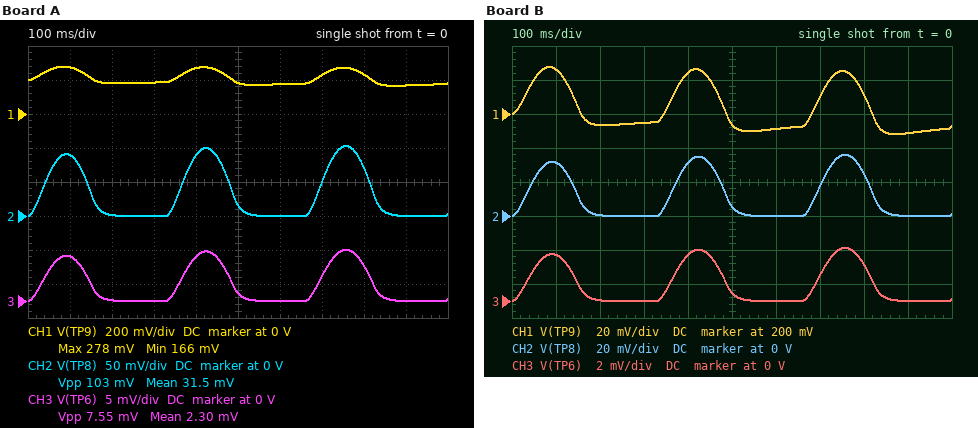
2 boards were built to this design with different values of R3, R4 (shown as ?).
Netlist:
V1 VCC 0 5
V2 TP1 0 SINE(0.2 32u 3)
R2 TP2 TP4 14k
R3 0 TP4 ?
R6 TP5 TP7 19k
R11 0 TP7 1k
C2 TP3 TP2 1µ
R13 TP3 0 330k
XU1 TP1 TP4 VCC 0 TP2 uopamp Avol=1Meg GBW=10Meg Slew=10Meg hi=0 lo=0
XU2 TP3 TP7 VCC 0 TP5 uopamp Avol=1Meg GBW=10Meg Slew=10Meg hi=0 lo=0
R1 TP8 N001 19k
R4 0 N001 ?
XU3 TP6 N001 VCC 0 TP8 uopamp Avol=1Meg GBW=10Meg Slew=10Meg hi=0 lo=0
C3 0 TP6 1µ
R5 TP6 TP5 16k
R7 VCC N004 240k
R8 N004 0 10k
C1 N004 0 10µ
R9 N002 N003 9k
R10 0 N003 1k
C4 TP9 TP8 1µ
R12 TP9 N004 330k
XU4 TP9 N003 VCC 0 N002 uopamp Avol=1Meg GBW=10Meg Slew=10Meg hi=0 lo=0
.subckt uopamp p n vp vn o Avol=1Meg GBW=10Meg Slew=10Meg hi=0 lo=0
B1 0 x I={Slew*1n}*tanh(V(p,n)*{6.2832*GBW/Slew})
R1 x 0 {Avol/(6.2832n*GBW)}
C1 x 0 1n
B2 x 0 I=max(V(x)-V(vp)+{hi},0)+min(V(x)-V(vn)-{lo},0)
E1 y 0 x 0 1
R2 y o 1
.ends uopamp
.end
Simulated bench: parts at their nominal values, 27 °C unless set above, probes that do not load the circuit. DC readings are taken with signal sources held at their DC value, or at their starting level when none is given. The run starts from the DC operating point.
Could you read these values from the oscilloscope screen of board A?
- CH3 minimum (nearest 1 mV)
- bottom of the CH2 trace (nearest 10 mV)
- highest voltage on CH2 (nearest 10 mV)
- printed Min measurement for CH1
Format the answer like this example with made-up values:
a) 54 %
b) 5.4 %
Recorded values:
a) 0 V
b) 0 V
c) 100 mV
d) 166 mV
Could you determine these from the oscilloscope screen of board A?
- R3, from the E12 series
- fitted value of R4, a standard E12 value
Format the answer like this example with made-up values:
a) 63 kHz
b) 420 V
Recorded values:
a) 1.2 kΩ
b) 1.5 kΩ
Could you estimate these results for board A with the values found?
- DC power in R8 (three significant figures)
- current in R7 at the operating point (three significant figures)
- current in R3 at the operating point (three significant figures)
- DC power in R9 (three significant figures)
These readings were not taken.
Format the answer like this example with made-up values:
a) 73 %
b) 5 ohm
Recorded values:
a) 4.00 µW
b) 20.0 µA
c) 167 µA
d) 360 µW
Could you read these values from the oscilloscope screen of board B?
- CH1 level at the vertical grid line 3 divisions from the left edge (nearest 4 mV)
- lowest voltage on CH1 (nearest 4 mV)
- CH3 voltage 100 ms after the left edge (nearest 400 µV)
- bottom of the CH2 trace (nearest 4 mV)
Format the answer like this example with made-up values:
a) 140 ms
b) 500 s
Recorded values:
a) 196 mV
b) 188 mV
c) 2.8 mV
d) 0 V
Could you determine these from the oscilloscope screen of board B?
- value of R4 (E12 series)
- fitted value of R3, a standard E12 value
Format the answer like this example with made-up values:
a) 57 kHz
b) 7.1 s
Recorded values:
a) 1.8 kΩ
b) 3.3 kΩ
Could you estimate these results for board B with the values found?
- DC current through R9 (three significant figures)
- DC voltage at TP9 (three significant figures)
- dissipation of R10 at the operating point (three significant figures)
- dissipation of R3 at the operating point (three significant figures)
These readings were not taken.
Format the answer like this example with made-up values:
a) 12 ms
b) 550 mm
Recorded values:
a) 200 µA
b) 200 mV
c) 40.0 µW
d) 12.1 µW
